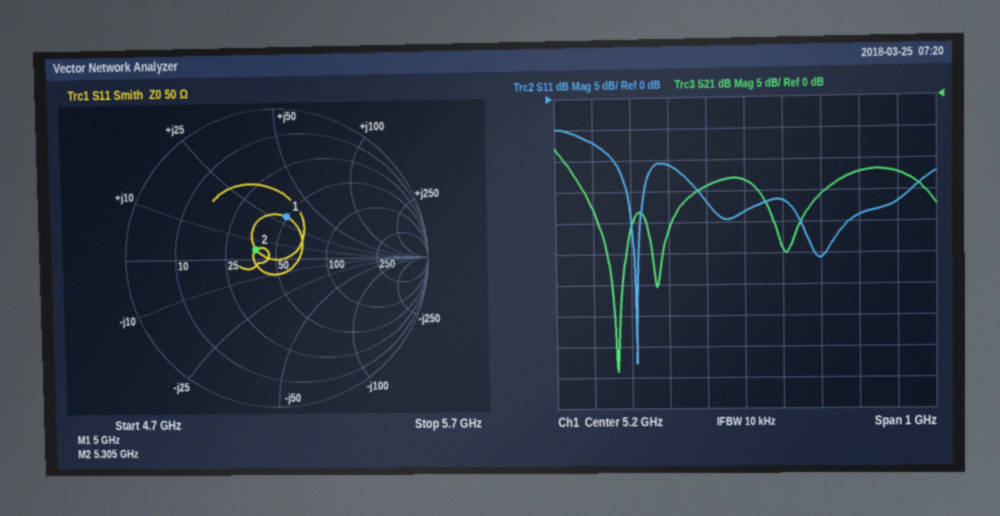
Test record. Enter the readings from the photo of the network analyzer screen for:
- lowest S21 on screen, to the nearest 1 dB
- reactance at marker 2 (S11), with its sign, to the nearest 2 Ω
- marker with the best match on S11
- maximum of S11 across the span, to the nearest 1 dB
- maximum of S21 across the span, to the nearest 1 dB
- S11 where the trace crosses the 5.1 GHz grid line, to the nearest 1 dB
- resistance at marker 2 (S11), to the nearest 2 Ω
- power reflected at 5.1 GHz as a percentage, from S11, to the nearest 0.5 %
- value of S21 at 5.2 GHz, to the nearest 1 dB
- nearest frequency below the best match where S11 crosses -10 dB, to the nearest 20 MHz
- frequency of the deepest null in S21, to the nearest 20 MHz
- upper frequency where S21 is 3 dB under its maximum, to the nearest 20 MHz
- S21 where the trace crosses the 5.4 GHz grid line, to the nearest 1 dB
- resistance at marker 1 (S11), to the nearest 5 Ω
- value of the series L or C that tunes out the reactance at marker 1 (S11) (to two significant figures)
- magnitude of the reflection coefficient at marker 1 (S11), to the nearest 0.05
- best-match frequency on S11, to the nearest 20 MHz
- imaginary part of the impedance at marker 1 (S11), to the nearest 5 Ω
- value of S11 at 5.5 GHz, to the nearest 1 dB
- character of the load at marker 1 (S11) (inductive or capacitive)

-44 dB
+4 Ω
marker 2
-5 dB
-8 dB
-17 dB
38 Ω
2.0 %
-13 dB
4.86 GHz
4.86 GHz
4.74 GHz
-16 dB
50 Ω
1.1 pF
0.30
4.92 GHz
+30 Ω
-19 dB
inductive
